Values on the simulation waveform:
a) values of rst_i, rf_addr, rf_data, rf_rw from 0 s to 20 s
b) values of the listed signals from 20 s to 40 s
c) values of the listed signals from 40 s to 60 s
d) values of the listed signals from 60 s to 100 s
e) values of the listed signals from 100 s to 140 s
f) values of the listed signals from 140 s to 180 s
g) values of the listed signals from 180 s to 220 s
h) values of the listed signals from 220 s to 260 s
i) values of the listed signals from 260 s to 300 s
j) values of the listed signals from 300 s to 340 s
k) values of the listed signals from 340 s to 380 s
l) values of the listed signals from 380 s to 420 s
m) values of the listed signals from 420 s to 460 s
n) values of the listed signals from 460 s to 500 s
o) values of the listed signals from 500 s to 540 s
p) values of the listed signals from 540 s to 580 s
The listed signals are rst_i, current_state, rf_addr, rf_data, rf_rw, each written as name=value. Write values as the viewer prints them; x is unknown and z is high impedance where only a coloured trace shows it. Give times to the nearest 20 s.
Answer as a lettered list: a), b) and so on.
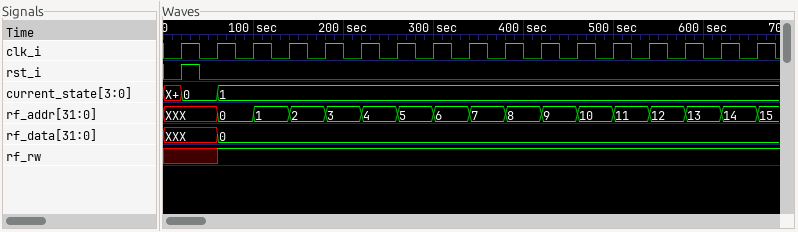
a) rst_i=0, rf_addr=XXX, rf_data=XXX, rf_rw=x
b) rst_i=1, current_state=0, rf_addr=XXX, rf_data=XXX, rf_rw=x
c) rst_i=0, current_state=0, rf_addr=XXX, rf_data=XXX, rf_rw=x
d) rst_i=0, current_state=1, rf_addr=0, rf_data=0, rf_rw=1
e) rst_i=0, current_state=1, rf_addr=1, rf_data=0, rf_rw=1
f) rst_i=0, current_state=1, rf_addr=2, rf_data=0, rf_rw=1
g) rst_i=0, current_state=1, rf_addr=3, rf_data=0, rf_rw=1
h) rst_i=0, current_state=1, rf_addr=4, rf_data=0, rf_rw=1
i) rst_i=0, current_state=1, rf_addr=5, rf_data=0, rf_rw=1
j) rst_i=0, current_state=1, rf_addr=6, rf_data=0, rf_rw=1
k) rst_i=0, current_state=1, rf_addr=7, rf_data=0, rf_rw=1
l) rst_i=0, current_state=1, rf_addr=8, rf_data=0, rf_rw=1
m) rst_i=0, current_state=1, rf_addr=9, rf_data=0, rf_rw=1
n) rst_i=0, current_state=1, rf_addr=10, rf_data=0, rf_rw=1
o) rst_i=0, current_state=1, rf_addr=11, rf_data=0, rf_rw=1
p) rst_i=0, current_state=1, rf_addr=12, rf_data=0, rf_rw=1
